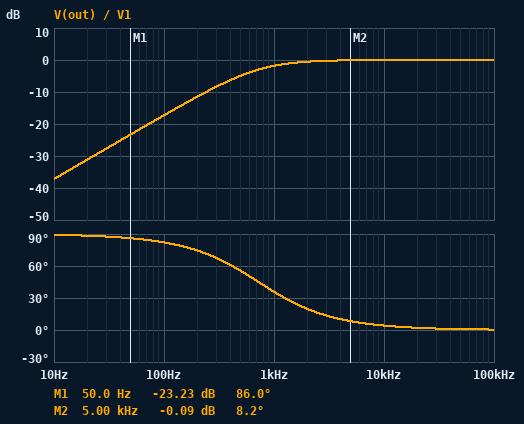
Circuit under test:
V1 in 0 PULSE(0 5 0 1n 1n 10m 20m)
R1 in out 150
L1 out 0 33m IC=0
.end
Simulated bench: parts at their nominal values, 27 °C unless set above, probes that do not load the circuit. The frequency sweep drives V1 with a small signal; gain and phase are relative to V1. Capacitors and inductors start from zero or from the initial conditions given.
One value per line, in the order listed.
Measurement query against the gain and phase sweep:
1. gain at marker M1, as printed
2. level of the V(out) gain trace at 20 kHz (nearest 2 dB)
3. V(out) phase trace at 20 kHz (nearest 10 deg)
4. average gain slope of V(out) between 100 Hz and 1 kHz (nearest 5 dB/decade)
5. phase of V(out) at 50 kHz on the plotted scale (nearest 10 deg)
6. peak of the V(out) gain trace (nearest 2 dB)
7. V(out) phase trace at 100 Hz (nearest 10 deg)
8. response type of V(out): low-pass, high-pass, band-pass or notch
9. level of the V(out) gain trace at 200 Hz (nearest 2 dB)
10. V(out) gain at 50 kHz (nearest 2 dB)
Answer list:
-23.23 dB
0 dB
0 deg
15 dB/decade
0 deg
0 dB
80 deg
high-pass
-12 dB
0 dB
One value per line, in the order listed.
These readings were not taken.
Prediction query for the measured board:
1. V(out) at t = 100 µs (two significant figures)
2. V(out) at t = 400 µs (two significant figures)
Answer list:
3.2 V
810 mV
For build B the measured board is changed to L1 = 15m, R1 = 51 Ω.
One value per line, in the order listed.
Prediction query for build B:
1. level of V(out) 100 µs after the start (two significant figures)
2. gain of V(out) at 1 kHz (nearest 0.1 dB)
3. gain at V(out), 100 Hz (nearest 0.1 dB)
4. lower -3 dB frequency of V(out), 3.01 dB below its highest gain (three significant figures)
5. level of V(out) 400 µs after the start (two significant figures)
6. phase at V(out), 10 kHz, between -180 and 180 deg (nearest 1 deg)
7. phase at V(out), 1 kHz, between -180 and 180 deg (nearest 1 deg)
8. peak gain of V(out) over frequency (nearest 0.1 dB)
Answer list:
3.6 V
-1.1 dB
-14.8 dB
541 Hz
1.3 V
3 deg
28 deg
0 dB
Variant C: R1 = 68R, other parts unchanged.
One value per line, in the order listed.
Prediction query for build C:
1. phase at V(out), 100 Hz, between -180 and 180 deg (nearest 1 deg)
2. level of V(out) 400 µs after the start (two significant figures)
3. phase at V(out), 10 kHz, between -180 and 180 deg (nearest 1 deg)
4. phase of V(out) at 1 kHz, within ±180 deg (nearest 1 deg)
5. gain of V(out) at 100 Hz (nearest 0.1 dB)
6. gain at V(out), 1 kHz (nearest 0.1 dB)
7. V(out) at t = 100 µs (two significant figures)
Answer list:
73 deg
2.2 V
2 deg
18 deg
-10.7 dB
-0.4 dB
4.1 V
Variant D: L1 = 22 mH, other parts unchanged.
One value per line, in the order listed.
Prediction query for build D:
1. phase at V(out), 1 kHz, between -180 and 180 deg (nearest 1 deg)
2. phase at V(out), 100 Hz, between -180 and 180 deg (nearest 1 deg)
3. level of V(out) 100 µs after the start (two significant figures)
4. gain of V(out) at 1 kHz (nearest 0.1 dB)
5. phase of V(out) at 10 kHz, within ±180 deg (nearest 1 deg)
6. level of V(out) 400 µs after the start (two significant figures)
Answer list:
47 deg
85 deg
2.5 V
-3.4 dB
6 deg
330 mV
